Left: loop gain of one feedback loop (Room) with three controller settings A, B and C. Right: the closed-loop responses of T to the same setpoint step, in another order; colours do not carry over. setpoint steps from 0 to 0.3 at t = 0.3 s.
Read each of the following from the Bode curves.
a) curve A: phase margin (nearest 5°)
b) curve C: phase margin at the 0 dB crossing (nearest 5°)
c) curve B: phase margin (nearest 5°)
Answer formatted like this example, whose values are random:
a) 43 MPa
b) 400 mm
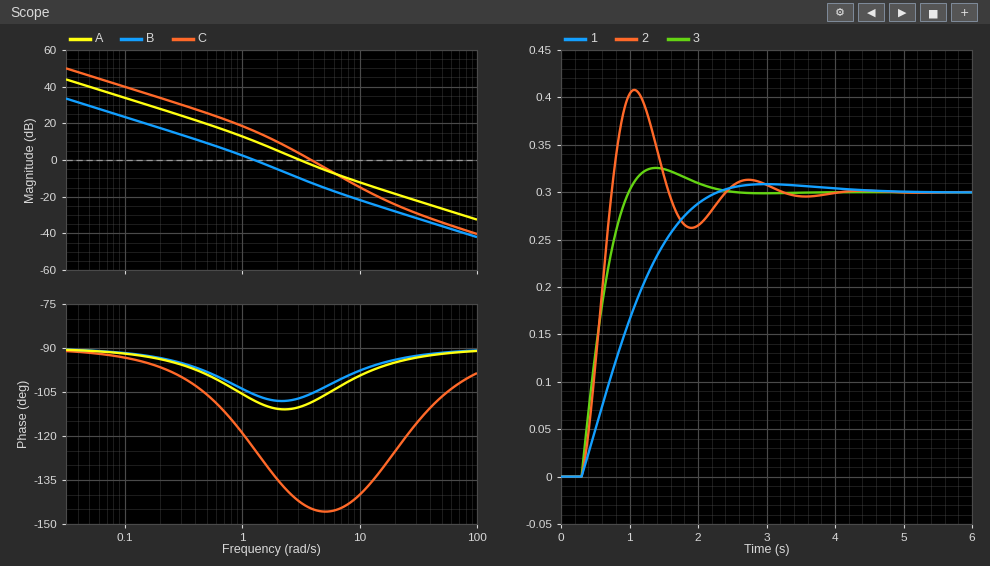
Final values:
a) 70°
b) 35°
c) 75°
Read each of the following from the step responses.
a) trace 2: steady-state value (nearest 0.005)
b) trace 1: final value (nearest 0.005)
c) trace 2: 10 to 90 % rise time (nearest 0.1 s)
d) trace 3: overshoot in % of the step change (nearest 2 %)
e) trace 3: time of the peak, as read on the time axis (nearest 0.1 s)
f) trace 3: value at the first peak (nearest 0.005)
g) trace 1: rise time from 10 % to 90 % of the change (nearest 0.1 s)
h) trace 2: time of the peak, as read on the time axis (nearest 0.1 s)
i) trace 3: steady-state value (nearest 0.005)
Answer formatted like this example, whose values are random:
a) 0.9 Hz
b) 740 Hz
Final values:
a) 0.300
b) 0.300
c) 0.3 s
d) 8 %
e) 1.4 s
f) 0.325
g) 1.3 s
h) 1.1 s
i) 0.300
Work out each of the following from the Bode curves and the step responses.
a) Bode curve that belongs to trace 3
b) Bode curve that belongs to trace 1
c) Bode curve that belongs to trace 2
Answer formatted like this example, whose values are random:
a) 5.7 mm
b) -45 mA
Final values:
a) A
b) B
c) C
